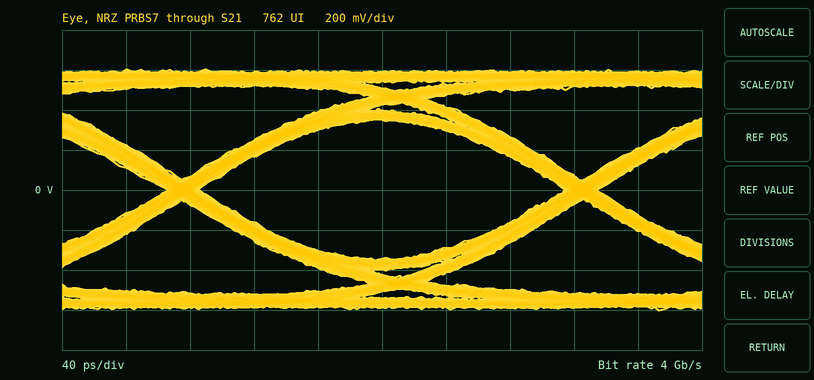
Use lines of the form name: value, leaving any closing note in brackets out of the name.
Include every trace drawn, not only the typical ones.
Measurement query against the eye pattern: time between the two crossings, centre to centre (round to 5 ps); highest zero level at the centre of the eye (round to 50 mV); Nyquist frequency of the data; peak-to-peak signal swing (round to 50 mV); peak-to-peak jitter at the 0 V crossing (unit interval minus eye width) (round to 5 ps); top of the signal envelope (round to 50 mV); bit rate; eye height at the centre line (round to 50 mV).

time between the two crossings, centre to centre: 250 ps
highest zero level at the centre of the eye: -350 mV
Nyquist frequency of the data: 2 GHz
peak-to-peak signal swing: 1.20 V
peak-to-peak jitter at the 0 V crossing (unit interval minus eye width): 20 ps
top of the signal envelope: 600 mV
bit rate: 4 Gb/s
eye height at the centre line: 700 mV
